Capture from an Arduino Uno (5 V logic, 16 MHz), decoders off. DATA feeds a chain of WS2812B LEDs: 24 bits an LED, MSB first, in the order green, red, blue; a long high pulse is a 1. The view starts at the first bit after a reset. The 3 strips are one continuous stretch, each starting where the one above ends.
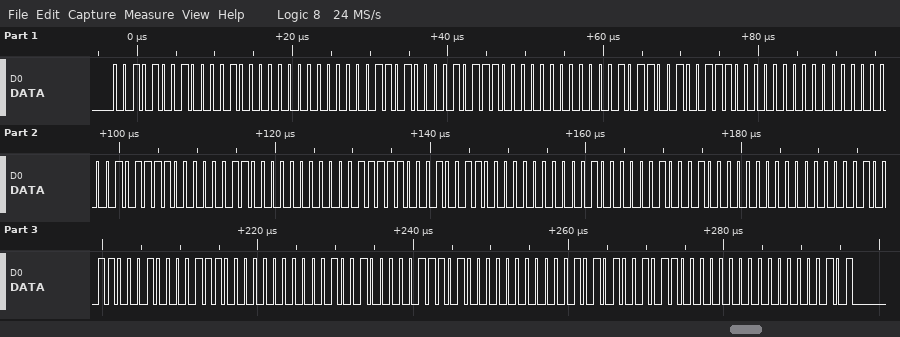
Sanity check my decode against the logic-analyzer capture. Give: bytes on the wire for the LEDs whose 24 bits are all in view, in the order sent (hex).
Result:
29 08 00 1A 17 00 0B 27 00 00 2F 03 00 1F 13 00 10 22 00 01 31 0E 00 24 1D 00 15 2C 00 05
